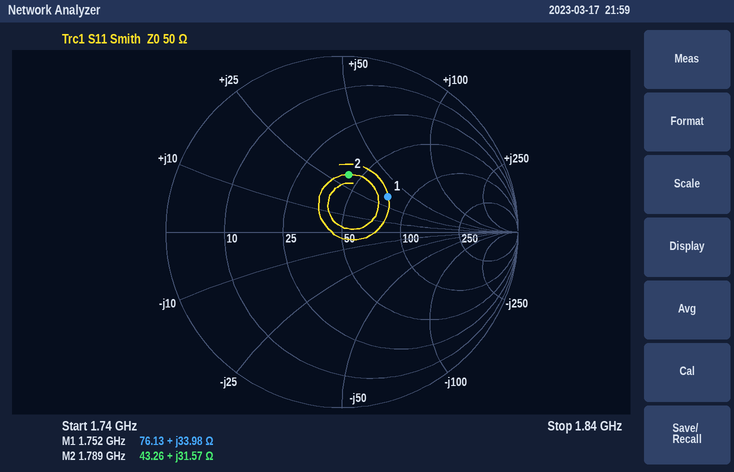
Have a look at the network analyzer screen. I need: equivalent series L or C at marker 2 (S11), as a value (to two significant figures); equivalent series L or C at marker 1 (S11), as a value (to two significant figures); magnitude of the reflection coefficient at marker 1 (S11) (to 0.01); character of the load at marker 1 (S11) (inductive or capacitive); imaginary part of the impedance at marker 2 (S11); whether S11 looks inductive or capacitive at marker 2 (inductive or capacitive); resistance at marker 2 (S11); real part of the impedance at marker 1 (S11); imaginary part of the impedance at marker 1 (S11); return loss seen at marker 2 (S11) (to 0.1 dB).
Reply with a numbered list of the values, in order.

1. 2.8 nH
2. 3.1 nH
3. 0.33
4. inductive
5. +31.57 Ω
6. inductive
7. 43.26 Ω
8. 76.13 Ω
9. +33.98 Ω
10. 9.7 dB
